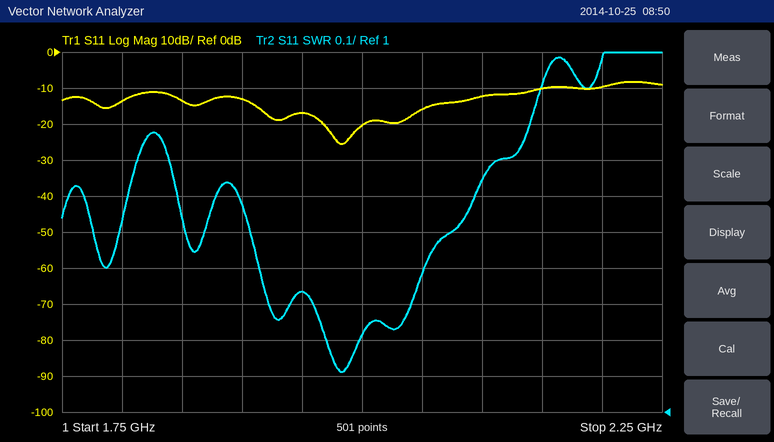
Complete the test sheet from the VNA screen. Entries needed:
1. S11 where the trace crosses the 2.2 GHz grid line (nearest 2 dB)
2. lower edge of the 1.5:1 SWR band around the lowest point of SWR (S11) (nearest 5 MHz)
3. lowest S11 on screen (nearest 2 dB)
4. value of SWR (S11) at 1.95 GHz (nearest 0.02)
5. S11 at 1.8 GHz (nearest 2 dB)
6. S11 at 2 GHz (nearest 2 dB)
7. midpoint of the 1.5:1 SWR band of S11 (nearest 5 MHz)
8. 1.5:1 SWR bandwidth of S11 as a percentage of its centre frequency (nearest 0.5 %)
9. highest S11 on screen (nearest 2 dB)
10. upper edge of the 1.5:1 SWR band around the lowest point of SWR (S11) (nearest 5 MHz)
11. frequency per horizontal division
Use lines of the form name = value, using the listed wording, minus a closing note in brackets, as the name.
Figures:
S11 where the trace crosses the 2.2 GHz grid line = -10 dB
lower edge of the 1.5:1 SWR band around the lowest point of SWR (S11) = 1.905 GHz
lowest S11 on screen = -26 dB
value of SWR (S11) at 1.95 GHz = 1.34
S11 at 1.8 GHz = -14 dB
S11 at 2 GHz = -20 dB
midpoint of the 1.5:1 SWR band of S11 = 1.990 GHz
1.5:1 SWR bandwidth of S11 as a percentage of its centre frequency = 8.5 %
highest S11 on screen = -8 dB
upper edge of the 1.5:1 SWR band around the lowest point of SWR (S11) = 2.075 GHz
frequency per horizontal division = 50 MHz
